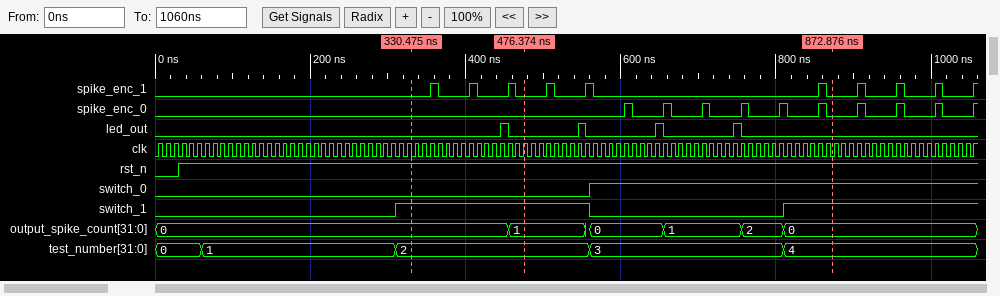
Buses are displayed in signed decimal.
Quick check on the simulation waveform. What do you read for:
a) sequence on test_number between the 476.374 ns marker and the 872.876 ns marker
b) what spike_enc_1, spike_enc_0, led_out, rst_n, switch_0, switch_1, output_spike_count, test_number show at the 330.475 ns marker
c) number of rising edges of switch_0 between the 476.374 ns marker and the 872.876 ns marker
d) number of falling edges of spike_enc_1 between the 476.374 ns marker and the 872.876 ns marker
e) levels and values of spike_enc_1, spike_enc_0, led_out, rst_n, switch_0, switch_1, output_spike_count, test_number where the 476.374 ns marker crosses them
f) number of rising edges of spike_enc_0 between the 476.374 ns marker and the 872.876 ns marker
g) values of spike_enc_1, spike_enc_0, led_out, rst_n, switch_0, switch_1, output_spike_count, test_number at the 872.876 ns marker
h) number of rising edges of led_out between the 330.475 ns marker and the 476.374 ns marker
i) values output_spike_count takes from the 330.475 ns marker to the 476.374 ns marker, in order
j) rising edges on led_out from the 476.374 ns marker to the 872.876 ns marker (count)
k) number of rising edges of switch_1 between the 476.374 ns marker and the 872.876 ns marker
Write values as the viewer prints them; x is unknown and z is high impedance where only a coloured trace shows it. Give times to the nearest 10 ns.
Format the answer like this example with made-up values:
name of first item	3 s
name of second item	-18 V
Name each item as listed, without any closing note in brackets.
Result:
sequence on test_number between the 476.374 ns marker and the 872.876 ns marker	2, 3, 4
what spike_enc_1, spike_enc_0, led_out, rst_n, switch_0, switch_1, output_spike_count, test_number show at the 330.475 ns marker	spike_enc_1=0, spike_enc_0=0, led_out=0, rst_n=1, switch_0=0, switch_1=1, output_spike_count=0, test_number=2
number of rising edges of switch_0 between the 476.374 ns marker and the 872.876 ns marker	1
number of falling edges of spike_enc_1 between the 476.374 ns marker and the 872.876 ns marker	3
levels and values of spike_enc_1, spike_enc_0, led_out, rst_n, switch_0, switch_1, output_spike_count, test_number where the 476.374 ns marker crosses them	spike_enc_1=0, spike_enc_0=0, led_out=0, rst_n=1, switch_0=0, switch_1=1, output_spike_count=1, test_number=2
number of rising edges of spike_enc_0 between the 476.374 ns marker and the 872.876 ns marker	6
values of spike_enc_1, spike_enc_0, led_out, rst_n, switch_0, switch_1, output_spike_count, test_number at the 872.876 ns marker	spike_enc_1=0, spike_enc_0=0, led_out=0, rst_n=1, switch_0=1, switch_1=1, output_spike_count=0, test_number=4
number of rising edges of led_out between the 330.475 ns marker and the 476.374 ns marker	1
values output_spike_count takes from the 330.475 ns marker to the 476.374 ns marker, in order	0, 1
rising edges on led_out from the 476.374 ns marker to the 872.876 ns marker	3
number of rising edges of switch_1 between the 476.374 ns marker and the 872.876 ns marker	1
